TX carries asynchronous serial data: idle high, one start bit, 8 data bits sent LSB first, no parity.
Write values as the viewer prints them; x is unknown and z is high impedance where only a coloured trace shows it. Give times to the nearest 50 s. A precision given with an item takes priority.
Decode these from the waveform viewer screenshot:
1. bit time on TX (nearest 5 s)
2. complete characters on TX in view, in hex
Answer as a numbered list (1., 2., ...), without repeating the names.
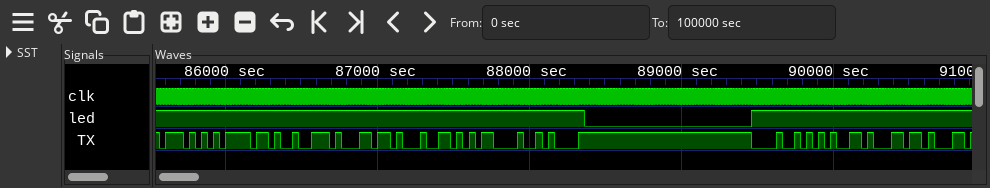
1. 40 s
2. 57, 6F, 72, 6C, 64, 0D, 0A, 48, 65, 6C
